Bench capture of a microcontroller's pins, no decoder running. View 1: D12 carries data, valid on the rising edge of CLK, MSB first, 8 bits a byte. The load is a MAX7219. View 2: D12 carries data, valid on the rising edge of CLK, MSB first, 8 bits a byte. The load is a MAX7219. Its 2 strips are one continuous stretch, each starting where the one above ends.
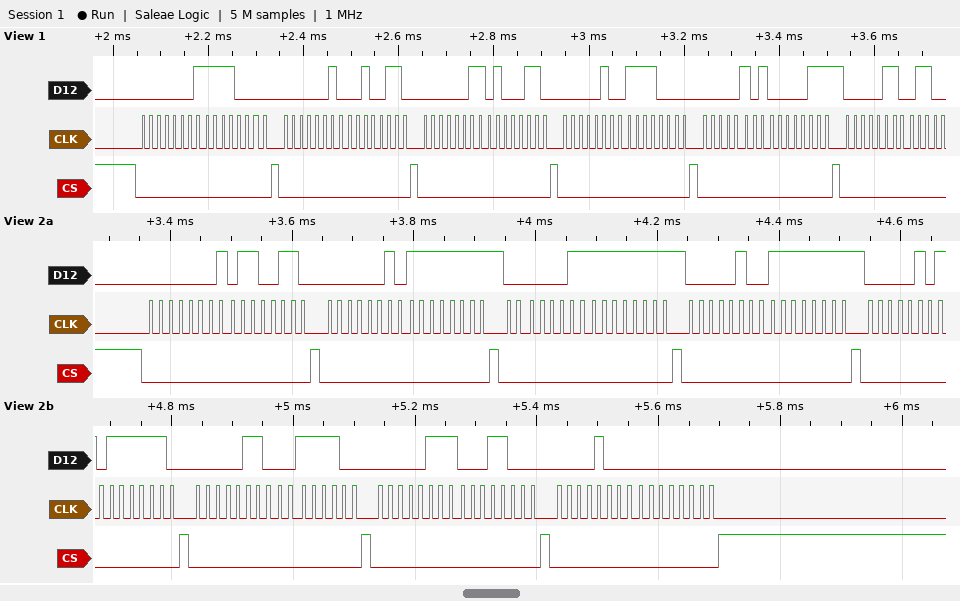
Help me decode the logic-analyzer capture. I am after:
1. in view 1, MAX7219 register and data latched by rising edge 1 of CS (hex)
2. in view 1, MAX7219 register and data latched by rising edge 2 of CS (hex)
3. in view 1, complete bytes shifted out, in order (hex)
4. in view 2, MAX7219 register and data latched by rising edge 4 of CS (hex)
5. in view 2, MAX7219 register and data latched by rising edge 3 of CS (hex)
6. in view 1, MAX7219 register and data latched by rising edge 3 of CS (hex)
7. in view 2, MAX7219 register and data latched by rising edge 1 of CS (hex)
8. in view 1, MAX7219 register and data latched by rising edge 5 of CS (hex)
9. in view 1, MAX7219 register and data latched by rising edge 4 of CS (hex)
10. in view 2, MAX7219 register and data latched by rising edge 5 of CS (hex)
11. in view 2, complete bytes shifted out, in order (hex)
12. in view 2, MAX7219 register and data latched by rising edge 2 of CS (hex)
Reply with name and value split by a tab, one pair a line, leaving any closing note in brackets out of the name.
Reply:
in view 1, MAX7219 register and data latched by rising edge 1 of CS	register 0x1, data 0xF0
in view 1, MAX7219 register and data latched by rising edge 2 of CS	register 0x2, data 0x26
in view 1, complete bytes shifted out, in order	01 F0 02 26 03 46 04 F0 05 07 06
in view 2, MAX7219 register and data latched by rising edge 4 of CS	register 0x4, data 0xFF
in view 2, MAX7219 register and data latched by rising edge 3 of CS	register 0x3, data 0xFF
in view 1, MAX7219 register and data latched by rising edge 3 of CS	register 0x3, data 0x46
in view 2, MAX7219 register and data latched by rising edge 1 of CS	register 0x1, data 0x66
in view 1, MAX7219 register and data latched by rising edge 5 of CS	register 0x5, data 0x07
in view 1, MAX7219 register and data latched by rising edge 4 of CS	register 0x4, data 0xF0
in view 2, MAX7219 register and data latched by rising edge 5 of CS	register 0x5, data 0x7E
in view 2, complete bytes shifted out, in order	0x01 0x66 0x02 0xFF 0x03 0xFF 0x04 0xFF 0x05 0x7E 0x06 0x3C 0x07 0x18 0x08 0x00
in view 2, MAX7219 register and data latched by rising edge 2 of CS	register 0x2, data 0xFF
